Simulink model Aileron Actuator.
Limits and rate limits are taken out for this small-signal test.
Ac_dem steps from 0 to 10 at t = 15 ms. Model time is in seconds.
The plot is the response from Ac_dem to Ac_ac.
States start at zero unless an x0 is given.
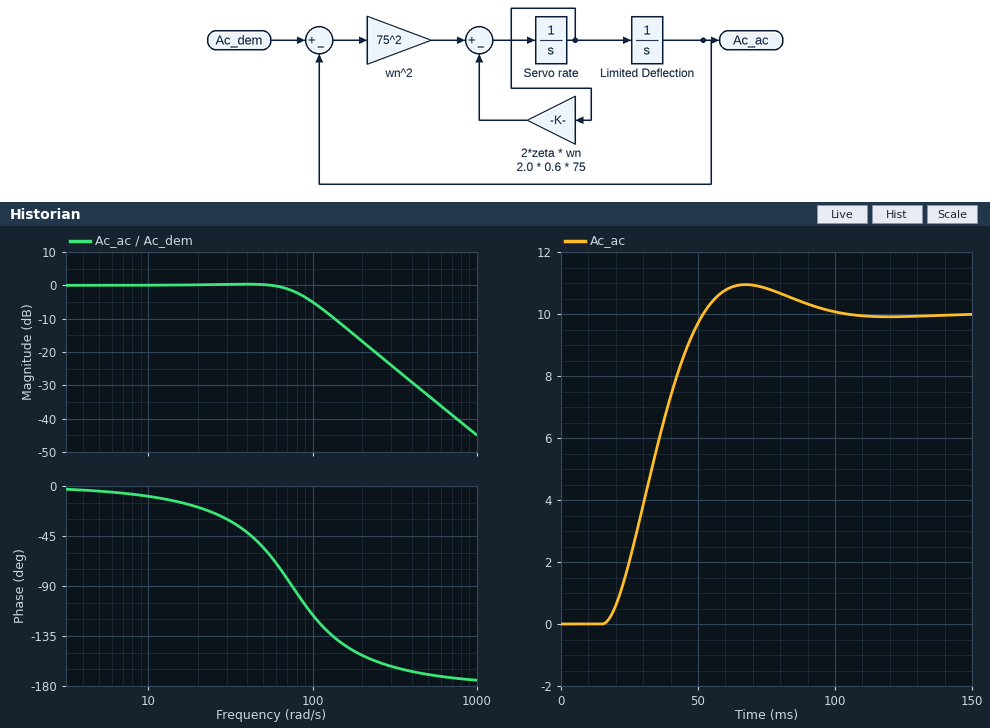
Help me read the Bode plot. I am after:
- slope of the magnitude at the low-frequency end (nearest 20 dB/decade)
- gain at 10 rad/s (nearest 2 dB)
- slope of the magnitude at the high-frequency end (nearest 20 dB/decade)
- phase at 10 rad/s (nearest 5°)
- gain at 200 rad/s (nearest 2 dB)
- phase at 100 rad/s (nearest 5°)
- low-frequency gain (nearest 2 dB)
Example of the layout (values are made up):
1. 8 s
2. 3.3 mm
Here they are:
1. 0 dB/decade
2. 0 dB
3. -40 dB/decade
4. -10°
5. -16 dB
6. -115°
7. 0 dB
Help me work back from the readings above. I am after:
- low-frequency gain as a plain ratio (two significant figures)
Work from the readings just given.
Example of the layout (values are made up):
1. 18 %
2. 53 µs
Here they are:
1. 1.0
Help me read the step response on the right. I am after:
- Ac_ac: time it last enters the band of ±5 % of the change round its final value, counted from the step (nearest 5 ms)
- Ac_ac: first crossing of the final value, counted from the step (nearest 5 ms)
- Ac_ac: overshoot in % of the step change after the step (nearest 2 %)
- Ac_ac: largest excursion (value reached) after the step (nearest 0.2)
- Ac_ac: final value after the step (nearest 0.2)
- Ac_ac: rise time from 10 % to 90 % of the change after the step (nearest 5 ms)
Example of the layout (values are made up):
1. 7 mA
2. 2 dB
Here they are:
1. 70 ms
2. 35 ms
3. 10 %
4. 11.0
5. 10.0
6. 25 ms
